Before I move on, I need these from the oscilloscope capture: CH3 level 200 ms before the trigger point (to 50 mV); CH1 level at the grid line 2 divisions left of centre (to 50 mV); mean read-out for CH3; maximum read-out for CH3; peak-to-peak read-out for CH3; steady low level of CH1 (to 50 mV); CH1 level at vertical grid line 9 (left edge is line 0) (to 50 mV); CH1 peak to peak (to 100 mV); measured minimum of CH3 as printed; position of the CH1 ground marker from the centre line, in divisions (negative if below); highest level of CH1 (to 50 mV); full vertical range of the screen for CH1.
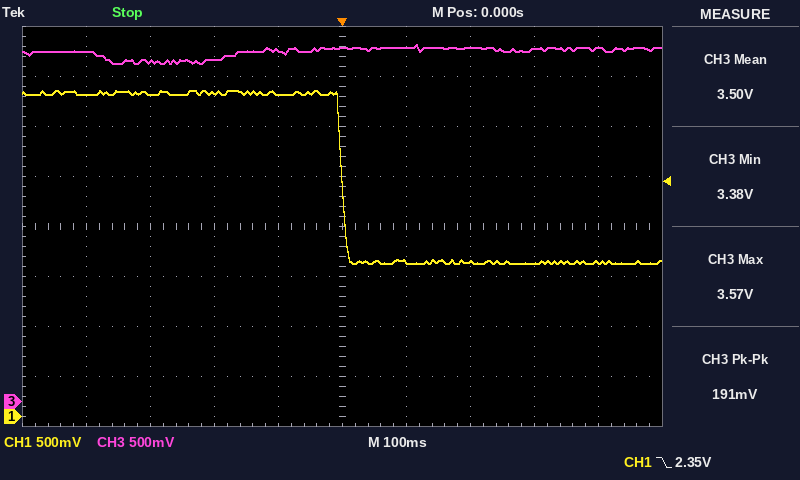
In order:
3.40 V
3.25 V
3.50 V
3.57 V
191 mV
1.55 V
1.55 V
1.70 V
3.38 V
-3.8 div
3.25 V
4 V
